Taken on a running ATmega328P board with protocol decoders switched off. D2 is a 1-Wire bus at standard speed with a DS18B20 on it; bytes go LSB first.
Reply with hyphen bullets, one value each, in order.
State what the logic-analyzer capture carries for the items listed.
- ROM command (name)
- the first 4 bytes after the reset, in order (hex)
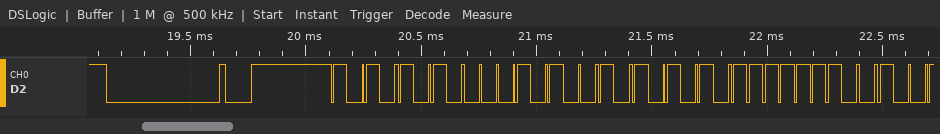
- Match ROM
- 55 28 55 7F
